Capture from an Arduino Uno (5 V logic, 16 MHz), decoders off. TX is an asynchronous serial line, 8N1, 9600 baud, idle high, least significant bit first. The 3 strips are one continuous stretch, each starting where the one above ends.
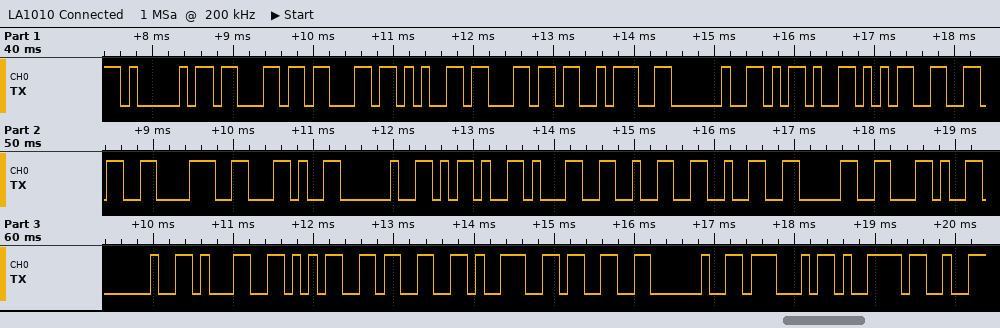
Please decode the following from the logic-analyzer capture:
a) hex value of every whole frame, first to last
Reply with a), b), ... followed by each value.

a) 41 63 63 65 6C 3A 20 2D 35 36 38 2C 20 2D 31 32 32 30 2C 20 31 35 33 39 33 20 47 79
